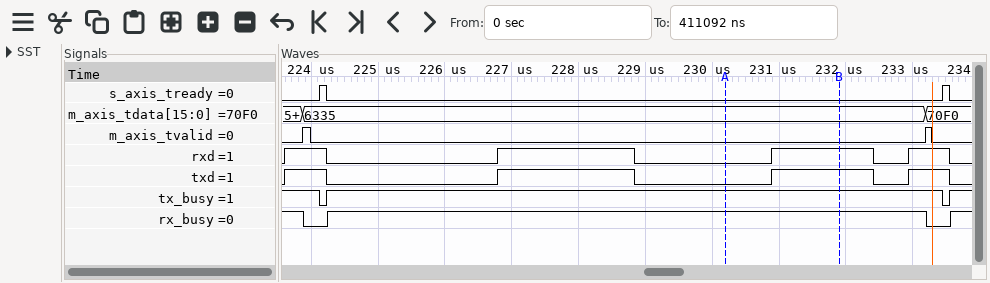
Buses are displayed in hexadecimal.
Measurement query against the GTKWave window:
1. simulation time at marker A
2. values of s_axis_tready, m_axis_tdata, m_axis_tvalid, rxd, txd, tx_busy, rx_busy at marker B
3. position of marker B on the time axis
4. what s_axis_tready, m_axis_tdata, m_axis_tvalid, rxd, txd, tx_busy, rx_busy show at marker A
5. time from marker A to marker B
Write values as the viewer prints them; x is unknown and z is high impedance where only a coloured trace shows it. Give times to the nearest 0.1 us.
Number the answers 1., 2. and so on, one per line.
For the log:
1. 230.2 us
2. s_axis_tready=0, m_axis_tdata=6335, m_axis_tvalid=0, rxd=1, txd=1, tx_busy=1, rx_busy=1
3. 231.9 us
4. s_axis_tready=0, m_axis_tdata=6335, m_axis_tvalid=0, rxd=0, txd=0, tx_busy=1, rx_busy=1
5. 1.7 us
